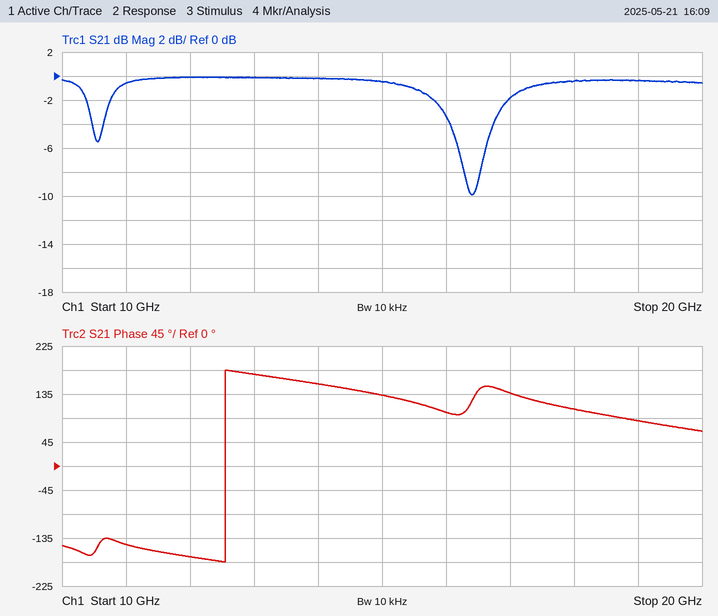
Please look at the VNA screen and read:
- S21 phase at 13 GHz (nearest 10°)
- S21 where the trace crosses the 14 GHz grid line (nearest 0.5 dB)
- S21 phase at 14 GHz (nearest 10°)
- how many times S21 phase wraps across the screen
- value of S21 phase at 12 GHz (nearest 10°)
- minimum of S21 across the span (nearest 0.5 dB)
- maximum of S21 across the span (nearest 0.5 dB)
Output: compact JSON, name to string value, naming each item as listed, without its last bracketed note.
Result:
{"S21 phase at 13 GHz": "170°", "S21 where the trace crosses the 14 GHz grid line": "0.0 dB", "S21 phase at 14 GHz": "150°", "how many times S21 phase wraps across the screen": "1", "value of S21 phase at 12 GHz": "-170°", "minimum of S21 across the span": "-10.0 dB", "maximum of S21 across the span": "0.0 dB"}
